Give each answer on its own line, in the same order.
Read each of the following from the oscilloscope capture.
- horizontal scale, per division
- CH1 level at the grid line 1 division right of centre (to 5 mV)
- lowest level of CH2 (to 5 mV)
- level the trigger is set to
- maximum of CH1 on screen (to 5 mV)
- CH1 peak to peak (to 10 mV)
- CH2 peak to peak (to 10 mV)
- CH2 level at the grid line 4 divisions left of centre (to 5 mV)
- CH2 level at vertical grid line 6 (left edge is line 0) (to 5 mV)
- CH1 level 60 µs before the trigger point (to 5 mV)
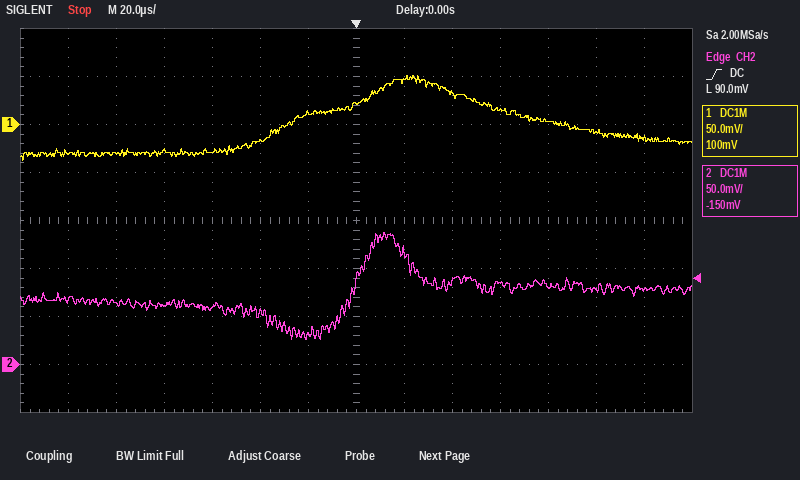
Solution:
20 µs
45 mV
25 mV
90.0 mV
50 mV
90 mV
110 mV
60 mV
30 mV
-30 mV
